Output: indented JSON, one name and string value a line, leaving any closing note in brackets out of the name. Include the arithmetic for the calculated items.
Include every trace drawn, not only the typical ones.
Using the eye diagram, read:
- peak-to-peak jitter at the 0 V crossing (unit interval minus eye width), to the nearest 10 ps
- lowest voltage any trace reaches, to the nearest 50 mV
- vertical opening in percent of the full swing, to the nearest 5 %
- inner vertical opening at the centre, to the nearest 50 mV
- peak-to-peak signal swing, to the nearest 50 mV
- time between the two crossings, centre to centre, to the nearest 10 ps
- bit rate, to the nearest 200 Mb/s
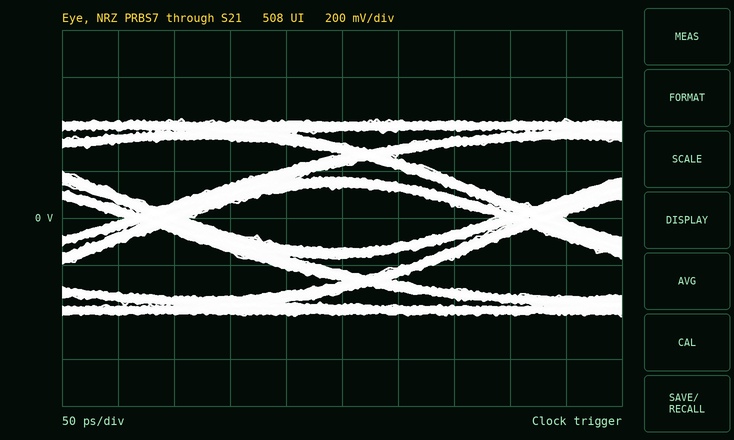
{
  "peak-to-peak jitter at the 0 V crossing (unit interval minus eye width), to the nearest 10 ps": "60 ps",
  "lowest voltage any trace reaches, to the nearest 50 mV": "-400 mV",
  "vertical opening in percent of the full swing, to the nearest 5 %": "250 mV / 850 mV ≈ 29.4 %, so 30 % to the nearest 5 %",
  "inner vertical opening at the centre, to the nearest 50 mV": "250 mV",
  "peak-to-peak signal swing, to the nearest 50 mV": "850 mV",
  "time between the two crossings, centre to centre, to the nearest 10 ps": "330 ps",
  "bit rate, to the nearest 200 Mb/s": "3.0 Gb/s"
}
